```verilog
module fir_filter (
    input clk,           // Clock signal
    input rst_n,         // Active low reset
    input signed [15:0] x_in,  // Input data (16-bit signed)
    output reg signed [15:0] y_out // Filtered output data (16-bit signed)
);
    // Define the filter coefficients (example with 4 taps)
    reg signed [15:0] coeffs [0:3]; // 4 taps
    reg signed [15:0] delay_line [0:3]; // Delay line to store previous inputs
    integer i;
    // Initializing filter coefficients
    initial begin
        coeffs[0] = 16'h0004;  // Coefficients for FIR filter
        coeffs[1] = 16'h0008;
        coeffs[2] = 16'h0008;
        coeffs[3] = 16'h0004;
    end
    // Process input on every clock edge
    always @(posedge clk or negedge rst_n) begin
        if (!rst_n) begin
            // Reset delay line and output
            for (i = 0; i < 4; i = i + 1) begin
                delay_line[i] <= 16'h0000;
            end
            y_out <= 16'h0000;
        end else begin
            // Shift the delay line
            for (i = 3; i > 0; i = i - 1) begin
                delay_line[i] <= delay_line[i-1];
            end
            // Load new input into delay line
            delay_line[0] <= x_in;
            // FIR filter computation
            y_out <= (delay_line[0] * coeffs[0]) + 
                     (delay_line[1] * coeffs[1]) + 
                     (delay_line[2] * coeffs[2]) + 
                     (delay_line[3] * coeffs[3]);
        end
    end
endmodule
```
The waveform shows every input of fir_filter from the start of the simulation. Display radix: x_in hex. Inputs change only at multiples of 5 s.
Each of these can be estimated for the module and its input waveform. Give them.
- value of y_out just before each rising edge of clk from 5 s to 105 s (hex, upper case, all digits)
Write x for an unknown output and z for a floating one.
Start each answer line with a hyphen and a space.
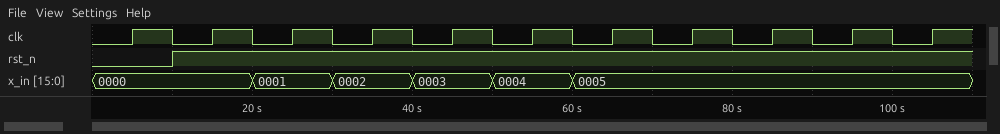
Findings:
- 0000, 0000, 0000, 0000, 0004, 0010, 0024, 003C, 0054, 0068, 0074
